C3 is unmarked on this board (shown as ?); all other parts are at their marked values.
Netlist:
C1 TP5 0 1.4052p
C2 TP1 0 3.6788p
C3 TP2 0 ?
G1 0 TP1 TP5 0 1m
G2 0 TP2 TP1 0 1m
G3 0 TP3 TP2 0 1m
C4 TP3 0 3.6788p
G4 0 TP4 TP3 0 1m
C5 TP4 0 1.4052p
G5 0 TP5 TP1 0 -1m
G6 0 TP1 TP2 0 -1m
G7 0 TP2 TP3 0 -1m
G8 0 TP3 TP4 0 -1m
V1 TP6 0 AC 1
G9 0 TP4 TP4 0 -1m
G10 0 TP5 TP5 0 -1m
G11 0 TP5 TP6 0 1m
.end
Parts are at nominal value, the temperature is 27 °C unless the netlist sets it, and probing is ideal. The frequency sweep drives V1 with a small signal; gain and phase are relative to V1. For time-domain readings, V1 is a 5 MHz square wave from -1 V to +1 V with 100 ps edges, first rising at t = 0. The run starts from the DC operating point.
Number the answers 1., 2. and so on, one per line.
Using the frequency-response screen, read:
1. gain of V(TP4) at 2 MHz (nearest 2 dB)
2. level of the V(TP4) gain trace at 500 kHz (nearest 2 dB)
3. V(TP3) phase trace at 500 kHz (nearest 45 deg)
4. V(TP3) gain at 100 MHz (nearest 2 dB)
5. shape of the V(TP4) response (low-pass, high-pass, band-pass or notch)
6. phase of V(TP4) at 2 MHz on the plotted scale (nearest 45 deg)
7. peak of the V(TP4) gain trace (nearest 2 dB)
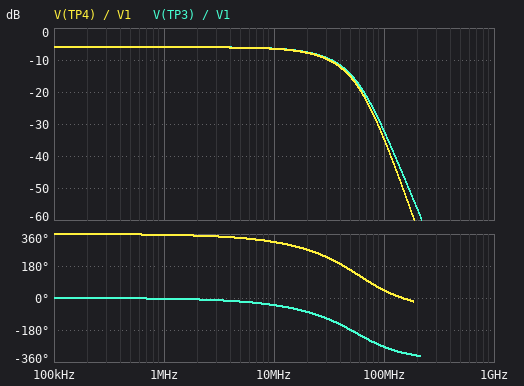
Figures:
1. -6 dB
2. -6 dB
3. 0 deg
4. -32 dB
5. low-pass
6. 360 deg
7. -6 dB
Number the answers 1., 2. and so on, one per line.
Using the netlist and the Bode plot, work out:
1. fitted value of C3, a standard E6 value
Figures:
1. 15 pF
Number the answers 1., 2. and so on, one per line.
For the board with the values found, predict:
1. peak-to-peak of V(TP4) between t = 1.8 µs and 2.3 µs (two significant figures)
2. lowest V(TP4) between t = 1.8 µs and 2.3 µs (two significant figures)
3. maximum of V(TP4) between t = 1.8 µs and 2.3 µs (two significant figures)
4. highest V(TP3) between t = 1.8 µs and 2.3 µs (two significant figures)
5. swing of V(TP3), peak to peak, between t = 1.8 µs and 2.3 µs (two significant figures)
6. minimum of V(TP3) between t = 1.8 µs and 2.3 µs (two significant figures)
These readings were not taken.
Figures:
1. 1.0 V
2. -500 mV
3. 500 mV
4. 500 mV
5. 1.0 V
6. -500 mV
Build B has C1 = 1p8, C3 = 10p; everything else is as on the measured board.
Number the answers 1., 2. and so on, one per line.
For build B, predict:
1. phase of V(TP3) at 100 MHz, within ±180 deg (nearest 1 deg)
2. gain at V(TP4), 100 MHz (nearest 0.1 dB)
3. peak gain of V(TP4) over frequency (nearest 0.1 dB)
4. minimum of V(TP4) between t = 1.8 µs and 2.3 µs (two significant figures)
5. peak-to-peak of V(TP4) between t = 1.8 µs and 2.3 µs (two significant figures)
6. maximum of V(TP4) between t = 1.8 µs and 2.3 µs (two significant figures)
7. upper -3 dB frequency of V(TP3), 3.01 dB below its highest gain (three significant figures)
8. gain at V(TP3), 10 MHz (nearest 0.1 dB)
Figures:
1. 75 deg
2. -31.5 dB
3. -6.0 dB
4. -540 mV
5. 1.1 V
6. 540 mV
7. 45.5 MHz
8. -6.1 dB
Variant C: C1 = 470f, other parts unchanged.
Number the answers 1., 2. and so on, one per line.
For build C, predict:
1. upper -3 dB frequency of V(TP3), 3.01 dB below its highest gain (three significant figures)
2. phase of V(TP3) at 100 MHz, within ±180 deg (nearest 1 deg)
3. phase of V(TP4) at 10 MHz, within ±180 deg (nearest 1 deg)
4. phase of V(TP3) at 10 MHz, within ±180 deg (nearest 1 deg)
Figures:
1. 27.1 MHz
2. 117 deg
3. -44 deg
4. -39 deg
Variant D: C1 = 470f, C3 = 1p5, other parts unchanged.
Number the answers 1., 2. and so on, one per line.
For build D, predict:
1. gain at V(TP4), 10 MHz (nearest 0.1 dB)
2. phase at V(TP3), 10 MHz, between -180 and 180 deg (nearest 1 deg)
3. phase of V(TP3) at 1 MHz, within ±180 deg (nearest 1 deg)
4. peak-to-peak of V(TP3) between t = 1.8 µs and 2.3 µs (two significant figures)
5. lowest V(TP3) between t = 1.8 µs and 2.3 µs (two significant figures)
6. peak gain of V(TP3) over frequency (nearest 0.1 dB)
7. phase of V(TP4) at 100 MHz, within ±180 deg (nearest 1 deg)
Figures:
1. -6.1 dB
2. -14 deg
3. -1 deg
4. 1.3 V
5. -650 mV
6. -3.6 dB
7. 158 deg
